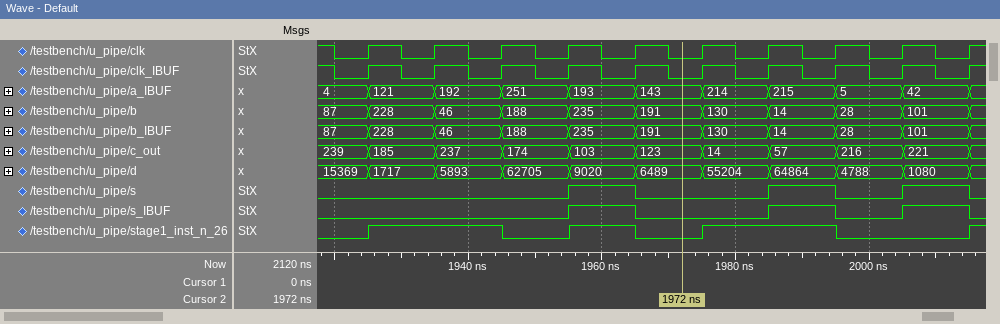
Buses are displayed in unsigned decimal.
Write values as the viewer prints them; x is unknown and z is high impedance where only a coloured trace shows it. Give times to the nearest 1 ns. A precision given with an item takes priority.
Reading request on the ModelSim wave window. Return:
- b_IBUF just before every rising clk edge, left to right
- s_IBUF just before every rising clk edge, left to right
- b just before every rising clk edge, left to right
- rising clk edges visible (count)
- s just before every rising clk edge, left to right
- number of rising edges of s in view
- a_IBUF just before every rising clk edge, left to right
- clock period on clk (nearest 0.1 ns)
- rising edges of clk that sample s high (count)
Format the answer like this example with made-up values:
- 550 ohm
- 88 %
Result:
- 87, 228, 46, 188, 235, 191, 130, 14, 28, 101
- 0 0 0 0 1 0 0 1 0 1
- 87, 228, 46, 188, 235, 191, 130, 14, 28, 101
- 10
- 0 0 0 0 1 0 0 1 0 1
- 3
- 4, 121, 192, 251, 193, 143, 214, 215, 5, 42
- 10 ns
- 3
